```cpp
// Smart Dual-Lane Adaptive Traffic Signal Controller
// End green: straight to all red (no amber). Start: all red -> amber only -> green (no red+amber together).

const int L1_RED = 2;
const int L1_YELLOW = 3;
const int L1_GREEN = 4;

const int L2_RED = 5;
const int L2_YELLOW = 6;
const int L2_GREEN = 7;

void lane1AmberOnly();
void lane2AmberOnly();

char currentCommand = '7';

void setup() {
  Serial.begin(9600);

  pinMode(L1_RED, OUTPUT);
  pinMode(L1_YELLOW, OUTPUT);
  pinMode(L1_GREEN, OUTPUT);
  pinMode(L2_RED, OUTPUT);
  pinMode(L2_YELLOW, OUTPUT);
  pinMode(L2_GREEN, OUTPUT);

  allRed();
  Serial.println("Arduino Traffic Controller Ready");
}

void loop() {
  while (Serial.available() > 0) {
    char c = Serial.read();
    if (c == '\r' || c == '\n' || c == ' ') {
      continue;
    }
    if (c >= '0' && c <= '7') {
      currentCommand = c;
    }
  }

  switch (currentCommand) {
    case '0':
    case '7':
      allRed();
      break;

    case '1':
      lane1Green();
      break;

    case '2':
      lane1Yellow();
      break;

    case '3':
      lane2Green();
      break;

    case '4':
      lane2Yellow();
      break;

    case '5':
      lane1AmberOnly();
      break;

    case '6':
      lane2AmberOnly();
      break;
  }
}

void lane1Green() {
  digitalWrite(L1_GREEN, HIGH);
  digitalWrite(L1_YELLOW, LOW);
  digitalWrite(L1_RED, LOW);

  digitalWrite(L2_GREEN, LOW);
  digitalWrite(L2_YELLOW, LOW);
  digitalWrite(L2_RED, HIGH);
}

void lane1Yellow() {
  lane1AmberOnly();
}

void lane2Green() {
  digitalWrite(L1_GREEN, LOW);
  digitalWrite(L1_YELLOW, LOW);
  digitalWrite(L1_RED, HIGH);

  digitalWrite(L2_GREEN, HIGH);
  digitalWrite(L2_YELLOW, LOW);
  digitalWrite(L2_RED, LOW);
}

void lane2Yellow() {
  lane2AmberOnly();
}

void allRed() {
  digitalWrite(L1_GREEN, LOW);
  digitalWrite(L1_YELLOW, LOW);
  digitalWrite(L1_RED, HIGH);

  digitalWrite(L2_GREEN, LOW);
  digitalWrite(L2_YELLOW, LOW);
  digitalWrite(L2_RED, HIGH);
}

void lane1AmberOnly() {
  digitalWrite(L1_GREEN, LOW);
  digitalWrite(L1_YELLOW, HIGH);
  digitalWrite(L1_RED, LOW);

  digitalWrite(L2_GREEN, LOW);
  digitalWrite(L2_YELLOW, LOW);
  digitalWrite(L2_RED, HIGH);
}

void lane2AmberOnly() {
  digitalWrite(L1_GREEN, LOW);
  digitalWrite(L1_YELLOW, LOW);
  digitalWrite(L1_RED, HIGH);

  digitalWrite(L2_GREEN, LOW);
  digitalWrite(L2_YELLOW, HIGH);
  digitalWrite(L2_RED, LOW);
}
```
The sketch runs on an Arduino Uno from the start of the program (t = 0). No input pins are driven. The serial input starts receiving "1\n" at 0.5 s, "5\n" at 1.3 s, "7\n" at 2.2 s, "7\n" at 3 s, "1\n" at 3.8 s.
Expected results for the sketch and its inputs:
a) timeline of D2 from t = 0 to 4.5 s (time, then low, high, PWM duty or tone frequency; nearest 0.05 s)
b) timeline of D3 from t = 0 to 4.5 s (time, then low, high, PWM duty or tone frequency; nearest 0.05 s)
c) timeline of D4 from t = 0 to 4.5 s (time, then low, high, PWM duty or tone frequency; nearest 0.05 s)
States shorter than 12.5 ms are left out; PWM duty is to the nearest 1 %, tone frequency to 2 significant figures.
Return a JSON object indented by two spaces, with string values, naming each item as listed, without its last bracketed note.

{
  "timeline of D2 from t = 0 to 4.5 s": "0 s high; 0.5 s low; 2.2 s high; 3.8 s low",
  "timeline of D3 from t = 0 to 4.5 s": "0 s low; 1.3 s high; 2.2 s low",
  "timeline of D4 from t = 0 to 4.5 s": "0 s low; 0.5 s high; 1.3 s low; 3.8 s high"
}
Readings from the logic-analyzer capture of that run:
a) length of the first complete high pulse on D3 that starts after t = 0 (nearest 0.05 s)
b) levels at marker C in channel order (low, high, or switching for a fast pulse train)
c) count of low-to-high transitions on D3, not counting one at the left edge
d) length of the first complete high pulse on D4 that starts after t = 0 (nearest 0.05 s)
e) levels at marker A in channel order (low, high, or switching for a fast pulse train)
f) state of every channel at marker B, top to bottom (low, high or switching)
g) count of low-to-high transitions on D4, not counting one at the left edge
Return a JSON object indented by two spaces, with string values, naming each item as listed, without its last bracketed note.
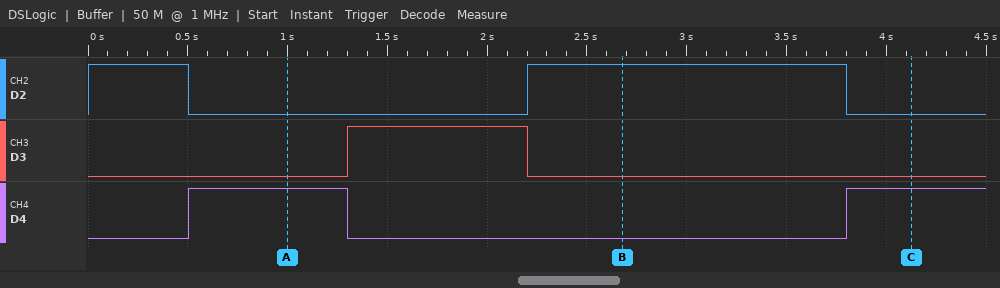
{
  "length of the first complete high pulse on D3 that starts after t = 0": "0.90 s",
  "levels at marker C in channel order": "D2 low, D3 low, D4 high",
  "count of low-to-high transitions on D3, not counting one at the left edge": "1",
  "length of the first complete high pulse on D4 that starts after t = 0": "0.80 s",
  "levels at marker A in channel order": "D2 low, D3 low, D4 high",
  "state of every channel at marker B, top to bottom": "D2 high, D3 low, D4 low",
  "count of low-to-high transitions on D4, not counting one at the left edge": "2"
}
